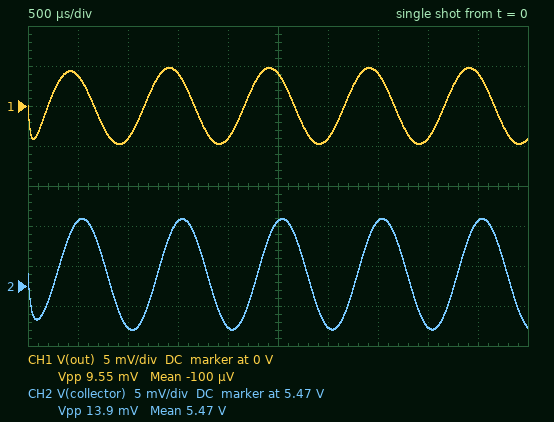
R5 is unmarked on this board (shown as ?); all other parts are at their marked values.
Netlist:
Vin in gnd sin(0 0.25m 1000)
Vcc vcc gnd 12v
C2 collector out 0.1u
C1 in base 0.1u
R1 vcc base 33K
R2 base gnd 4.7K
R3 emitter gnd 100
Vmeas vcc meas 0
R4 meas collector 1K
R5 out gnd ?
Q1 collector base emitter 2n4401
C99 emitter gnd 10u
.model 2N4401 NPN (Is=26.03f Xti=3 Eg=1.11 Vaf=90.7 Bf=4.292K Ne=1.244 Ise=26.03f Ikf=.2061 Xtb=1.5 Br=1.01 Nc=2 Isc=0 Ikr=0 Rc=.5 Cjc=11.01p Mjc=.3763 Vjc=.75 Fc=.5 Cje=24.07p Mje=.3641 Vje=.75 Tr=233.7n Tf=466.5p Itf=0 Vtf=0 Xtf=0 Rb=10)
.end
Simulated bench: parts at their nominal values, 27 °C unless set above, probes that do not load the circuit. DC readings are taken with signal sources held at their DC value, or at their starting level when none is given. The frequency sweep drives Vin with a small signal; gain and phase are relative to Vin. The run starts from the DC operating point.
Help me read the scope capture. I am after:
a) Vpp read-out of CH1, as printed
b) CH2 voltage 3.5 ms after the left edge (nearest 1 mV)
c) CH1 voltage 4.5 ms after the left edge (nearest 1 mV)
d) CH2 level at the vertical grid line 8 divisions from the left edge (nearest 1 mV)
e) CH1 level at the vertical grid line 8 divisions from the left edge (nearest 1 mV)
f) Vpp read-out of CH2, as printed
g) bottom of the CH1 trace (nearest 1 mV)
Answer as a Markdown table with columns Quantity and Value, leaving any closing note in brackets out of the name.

| Quantity | Value |
|---|---|
| Vpp read-out of CH1, as printed | 9.55 mV |
| CH2 voltage 3.5 ms after the left edge | 5.478 V |
| CH1 voltage 4.5 ms after the left edge | 4 mV |
| CH2 level at the vertical grid line 8 divisions from the left edge | 5.465 V |
| CH1 level at the vertical grid line 8 divisions from the left edge | -4 mV |
| Vpp read-out of CH2, as printed | 13.9 mV |
| bottom of the CH1 trace | -5 mV |
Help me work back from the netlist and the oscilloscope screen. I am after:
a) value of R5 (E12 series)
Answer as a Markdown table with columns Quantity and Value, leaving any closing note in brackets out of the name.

| Quantity | Value |
|---|---|
| value of R5 | 1.5 kΩ |
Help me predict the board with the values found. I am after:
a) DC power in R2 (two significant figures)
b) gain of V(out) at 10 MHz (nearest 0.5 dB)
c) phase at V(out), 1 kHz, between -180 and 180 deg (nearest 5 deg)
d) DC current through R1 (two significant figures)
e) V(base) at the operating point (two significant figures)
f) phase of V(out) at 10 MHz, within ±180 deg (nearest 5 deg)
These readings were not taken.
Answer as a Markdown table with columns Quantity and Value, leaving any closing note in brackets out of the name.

| Quantity | Value |
|---|---|
| DC power in R2 | 380 µW |
| gain of V(out) at 10 MHz | 41.0 dB |
| phase at V(out), 1 kHz, between -180 and 180 deg | -60 deg |
| DC current through R1 | 320 µA |
| V(base) at the operating point | 1.3 V |
| phase of V(out) at 10 MHz, within ±180 deg | 140 deg |
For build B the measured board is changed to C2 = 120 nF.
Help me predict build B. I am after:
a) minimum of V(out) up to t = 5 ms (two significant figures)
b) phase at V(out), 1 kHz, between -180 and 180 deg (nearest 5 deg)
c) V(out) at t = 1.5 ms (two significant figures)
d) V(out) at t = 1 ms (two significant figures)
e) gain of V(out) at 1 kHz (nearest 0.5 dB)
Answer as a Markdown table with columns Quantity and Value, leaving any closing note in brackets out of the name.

| Quantity | Value |
|---|---|
| minimum of V(out) up to t = 5 ms | -5.0 mV |
| phase at V(out), 1 kHz, between -180 and 180 deg | -65 deg |
| V(out) at t = 1.5 ms | 4.5 mV |
| V(out) at t = 1 ms | -4.5 mV |
| gain of V(out) at 1 kHz | 26.0 dB |
